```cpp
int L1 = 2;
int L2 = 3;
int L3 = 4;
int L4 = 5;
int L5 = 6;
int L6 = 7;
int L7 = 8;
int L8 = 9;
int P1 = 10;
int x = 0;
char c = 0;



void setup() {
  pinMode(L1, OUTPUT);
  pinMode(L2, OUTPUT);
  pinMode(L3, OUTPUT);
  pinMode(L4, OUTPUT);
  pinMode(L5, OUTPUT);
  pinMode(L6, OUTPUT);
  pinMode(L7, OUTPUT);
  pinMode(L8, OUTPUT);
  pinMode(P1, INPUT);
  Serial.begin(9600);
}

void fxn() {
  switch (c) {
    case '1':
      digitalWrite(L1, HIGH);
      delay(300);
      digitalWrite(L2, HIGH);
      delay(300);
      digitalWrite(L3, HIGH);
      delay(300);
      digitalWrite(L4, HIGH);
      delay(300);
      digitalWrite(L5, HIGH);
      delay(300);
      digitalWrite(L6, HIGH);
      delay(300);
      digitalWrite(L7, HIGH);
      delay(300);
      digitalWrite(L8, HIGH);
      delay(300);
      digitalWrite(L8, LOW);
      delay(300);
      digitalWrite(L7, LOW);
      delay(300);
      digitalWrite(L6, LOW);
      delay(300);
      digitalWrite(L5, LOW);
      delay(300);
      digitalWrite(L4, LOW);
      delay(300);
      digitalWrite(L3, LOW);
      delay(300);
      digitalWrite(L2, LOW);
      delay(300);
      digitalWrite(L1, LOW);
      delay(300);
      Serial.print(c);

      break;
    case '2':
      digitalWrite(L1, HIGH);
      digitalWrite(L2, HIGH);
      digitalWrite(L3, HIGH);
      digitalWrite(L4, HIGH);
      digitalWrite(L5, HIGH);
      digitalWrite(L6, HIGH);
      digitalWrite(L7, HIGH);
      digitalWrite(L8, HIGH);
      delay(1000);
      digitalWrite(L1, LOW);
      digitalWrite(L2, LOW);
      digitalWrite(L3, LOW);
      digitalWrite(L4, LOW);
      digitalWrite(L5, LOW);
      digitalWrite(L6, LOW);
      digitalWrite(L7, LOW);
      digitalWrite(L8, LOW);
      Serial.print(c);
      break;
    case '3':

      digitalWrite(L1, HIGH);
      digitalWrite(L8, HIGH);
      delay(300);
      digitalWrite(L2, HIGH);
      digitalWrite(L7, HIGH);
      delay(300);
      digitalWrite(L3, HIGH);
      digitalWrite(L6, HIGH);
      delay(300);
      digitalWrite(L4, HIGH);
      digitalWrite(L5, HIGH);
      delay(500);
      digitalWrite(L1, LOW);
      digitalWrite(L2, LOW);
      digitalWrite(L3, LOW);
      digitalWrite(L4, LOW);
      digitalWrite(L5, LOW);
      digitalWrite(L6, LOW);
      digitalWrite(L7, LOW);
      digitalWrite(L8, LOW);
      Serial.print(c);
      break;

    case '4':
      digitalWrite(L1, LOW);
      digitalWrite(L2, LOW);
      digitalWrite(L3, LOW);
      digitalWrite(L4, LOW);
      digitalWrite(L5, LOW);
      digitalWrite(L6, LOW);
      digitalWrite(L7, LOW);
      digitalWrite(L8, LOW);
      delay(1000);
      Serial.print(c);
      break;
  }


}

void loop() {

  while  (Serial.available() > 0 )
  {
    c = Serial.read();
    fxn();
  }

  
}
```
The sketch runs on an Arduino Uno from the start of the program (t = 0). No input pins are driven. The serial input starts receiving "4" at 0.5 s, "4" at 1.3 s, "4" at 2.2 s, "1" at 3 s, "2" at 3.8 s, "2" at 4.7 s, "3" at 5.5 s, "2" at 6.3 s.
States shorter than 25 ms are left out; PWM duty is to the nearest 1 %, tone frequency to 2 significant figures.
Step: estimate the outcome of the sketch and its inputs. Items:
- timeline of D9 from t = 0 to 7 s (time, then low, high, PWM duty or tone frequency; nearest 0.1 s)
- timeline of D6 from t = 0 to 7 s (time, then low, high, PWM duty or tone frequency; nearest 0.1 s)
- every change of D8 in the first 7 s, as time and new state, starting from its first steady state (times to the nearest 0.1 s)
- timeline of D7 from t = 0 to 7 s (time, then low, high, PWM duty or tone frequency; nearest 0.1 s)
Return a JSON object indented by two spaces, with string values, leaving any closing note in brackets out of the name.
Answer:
{
  "timeline of D9 from t = 0 to 7 s": "0 s low; 5.6 s high; 5.9 s low",
  "timeline of D6 from t = 0 to 7 s": "0 s low; 4.7 s high; 6.8 s low",
  "every change of D8 in the first 7 s, as time and new state, starting from its first steady state": "0 s low; 5.3 s high; 6.2 s low",
  "timeline of D7 from t = 0 to 7 s": "0 s low; 5 s high; 6.5 s low"
}
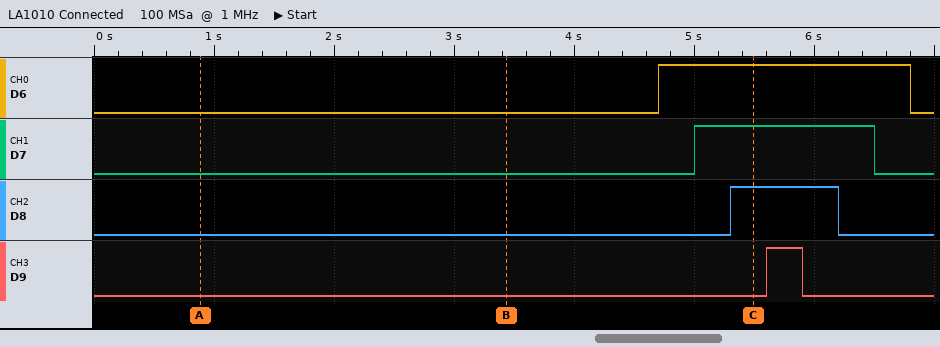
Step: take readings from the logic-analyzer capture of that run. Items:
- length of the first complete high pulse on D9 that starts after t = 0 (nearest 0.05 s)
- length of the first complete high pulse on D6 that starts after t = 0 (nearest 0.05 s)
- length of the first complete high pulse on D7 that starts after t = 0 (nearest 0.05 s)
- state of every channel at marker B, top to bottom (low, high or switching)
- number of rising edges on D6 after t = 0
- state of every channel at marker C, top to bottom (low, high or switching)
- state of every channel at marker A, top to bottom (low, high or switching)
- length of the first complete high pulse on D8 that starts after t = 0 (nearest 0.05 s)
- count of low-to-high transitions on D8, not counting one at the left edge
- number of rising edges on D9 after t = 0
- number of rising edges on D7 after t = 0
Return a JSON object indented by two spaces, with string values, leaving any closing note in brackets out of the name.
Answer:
{
  "length of the first complete high pulse on D9 that starts after t = 0": "0.30 s",
  "length of the first complete high pulse on D6 that starts after t = 0": "2.10 s",
  "length of the first complete high pulse on D7 that starts after t = 0": "1.50 s",
  "state of every channel at marker B, top to bottom": "D6 low, D7 low, D8 low, D9 low",
  "number of rising edges on D6 after t = 0": "1",
  "state of every channel at marker C, top to bottom": "D6 high, D7 high, D8 high, D9 low",
  "state of every channel at marker A, top to bottom": "D6 low, D7 low, D8 low, D9 low",
  "length of the first complete high pulse on D8 that starts after t = 0": "0.90 s",
  "count of low-to-high transitions on D8, not counting one at the left edge": "1",
  "number of rising edges on D9 after t = 0": "1",
  "number of rising edges on D7 after t = 0": "1"
}
